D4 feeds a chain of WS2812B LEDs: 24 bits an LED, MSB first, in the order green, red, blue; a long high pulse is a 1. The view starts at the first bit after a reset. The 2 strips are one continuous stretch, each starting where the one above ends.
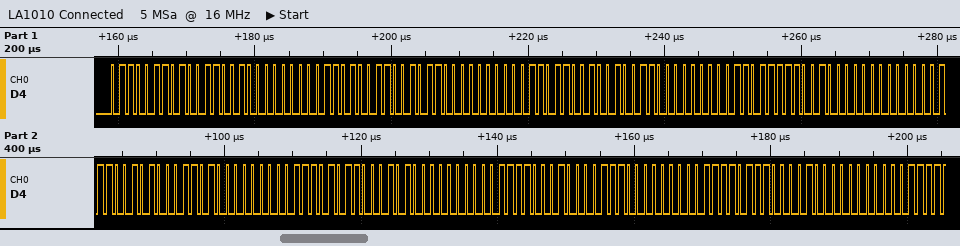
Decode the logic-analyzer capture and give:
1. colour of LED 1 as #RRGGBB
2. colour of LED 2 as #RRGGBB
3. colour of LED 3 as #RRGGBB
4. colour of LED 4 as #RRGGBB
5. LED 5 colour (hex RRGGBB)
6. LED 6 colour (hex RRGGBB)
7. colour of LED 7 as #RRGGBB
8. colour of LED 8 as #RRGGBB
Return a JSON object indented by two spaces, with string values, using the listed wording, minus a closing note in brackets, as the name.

{
  "colour of LED 1 as #RRGGBB": "#996600",
  "colour of LED 2 as #RRGGBB": "#966900",
  "colour of LED 3 as #RRGGBB": "#936C00",
  "colour of LED 4 as #RRGGBB": "#906F00",
  "LED 5 colour": "#8D7200",
  "LED 6 colour": "#8A7500",
  "colour of LED 7 as #RRGGBB": "#877800",
  "colour of LED 8 as #RRGGBB": "#847B00"
}
